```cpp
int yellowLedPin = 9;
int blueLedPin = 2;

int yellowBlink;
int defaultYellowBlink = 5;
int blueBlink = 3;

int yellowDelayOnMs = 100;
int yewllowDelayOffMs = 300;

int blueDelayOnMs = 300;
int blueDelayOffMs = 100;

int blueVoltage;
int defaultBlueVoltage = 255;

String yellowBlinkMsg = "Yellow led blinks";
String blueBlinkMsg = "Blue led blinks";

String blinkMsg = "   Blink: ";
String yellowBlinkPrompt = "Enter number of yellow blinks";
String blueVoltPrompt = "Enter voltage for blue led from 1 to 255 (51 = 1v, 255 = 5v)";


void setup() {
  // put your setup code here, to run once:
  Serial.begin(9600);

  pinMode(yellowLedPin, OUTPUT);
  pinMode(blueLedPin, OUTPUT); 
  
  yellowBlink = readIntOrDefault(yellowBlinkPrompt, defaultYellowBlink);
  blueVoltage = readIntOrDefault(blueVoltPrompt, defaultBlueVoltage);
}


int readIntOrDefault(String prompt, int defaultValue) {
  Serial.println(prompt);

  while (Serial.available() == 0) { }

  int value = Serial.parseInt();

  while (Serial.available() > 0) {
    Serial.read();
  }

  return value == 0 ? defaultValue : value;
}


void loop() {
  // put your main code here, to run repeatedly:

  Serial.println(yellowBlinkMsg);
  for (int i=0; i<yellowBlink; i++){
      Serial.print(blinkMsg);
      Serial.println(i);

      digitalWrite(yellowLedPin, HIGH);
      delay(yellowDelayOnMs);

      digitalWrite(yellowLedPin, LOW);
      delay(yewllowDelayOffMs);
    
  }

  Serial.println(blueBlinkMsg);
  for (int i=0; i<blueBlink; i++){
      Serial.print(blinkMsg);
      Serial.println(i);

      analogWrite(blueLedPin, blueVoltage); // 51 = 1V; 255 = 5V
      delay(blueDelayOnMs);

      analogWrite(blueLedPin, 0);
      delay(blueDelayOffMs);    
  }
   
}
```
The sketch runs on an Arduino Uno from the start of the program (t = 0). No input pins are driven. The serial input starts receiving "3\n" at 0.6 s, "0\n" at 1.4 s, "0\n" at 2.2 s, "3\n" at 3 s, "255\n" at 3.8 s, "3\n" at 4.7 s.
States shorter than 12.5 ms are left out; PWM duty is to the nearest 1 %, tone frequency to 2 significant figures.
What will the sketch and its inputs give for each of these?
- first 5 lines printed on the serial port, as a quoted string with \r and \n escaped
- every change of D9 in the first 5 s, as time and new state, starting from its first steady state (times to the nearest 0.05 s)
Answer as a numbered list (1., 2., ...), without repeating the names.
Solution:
1. "Enter number of yellow blinks\r\nEnter voltage for blue led from 1 to 255 (51 = 1v, 255 = 5v)\r\nYellow led blinks\r\n   Blink: 0\r\n   Blink: 1\r\n"
2. 0 s low; 1.4 s high; 1.5 s low; 1.8 s high; 1.9 s low; 2.2 s high; 2.3 s low; 3.8 s high; 3.9 s low; 4.2 s high; 4.3 s low; 4.6 s high; 4.7 s low
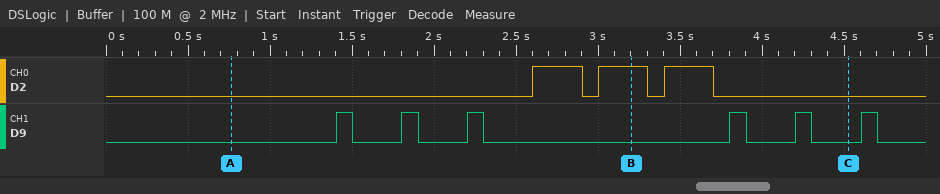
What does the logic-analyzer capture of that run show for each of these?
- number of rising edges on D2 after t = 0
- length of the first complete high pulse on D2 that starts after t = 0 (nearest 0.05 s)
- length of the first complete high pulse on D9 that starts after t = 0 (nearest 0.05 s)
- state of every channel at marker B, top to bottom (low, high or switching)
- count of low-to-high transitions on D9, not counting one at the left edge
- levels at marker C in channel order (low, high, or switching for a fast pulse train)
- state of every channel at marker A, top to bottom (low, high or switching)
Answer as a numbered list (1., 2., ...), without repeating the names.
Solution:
1. 3
2. 0.30 s
3. 0.10 s
4. D2 high, D9 low
5. 6
6. D2 low, D9 low
7. D2 low, D9 low
